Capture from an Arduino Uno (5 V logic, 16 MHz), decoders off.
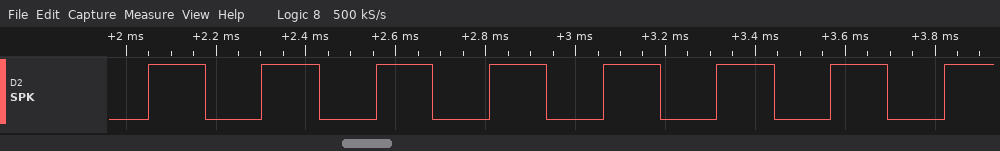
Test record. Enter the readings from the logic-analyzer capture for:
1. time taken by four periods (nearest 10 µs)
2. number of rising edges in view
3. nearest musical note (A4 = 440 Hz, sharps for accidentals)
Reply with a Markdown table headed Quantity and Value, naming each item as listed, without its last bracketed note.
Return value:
| Quantity | Value |
|---|---|
| time taken by four periods | 1010 µs |
| number of rising edges in view | 8 |
| nearest musical note | B7 |
